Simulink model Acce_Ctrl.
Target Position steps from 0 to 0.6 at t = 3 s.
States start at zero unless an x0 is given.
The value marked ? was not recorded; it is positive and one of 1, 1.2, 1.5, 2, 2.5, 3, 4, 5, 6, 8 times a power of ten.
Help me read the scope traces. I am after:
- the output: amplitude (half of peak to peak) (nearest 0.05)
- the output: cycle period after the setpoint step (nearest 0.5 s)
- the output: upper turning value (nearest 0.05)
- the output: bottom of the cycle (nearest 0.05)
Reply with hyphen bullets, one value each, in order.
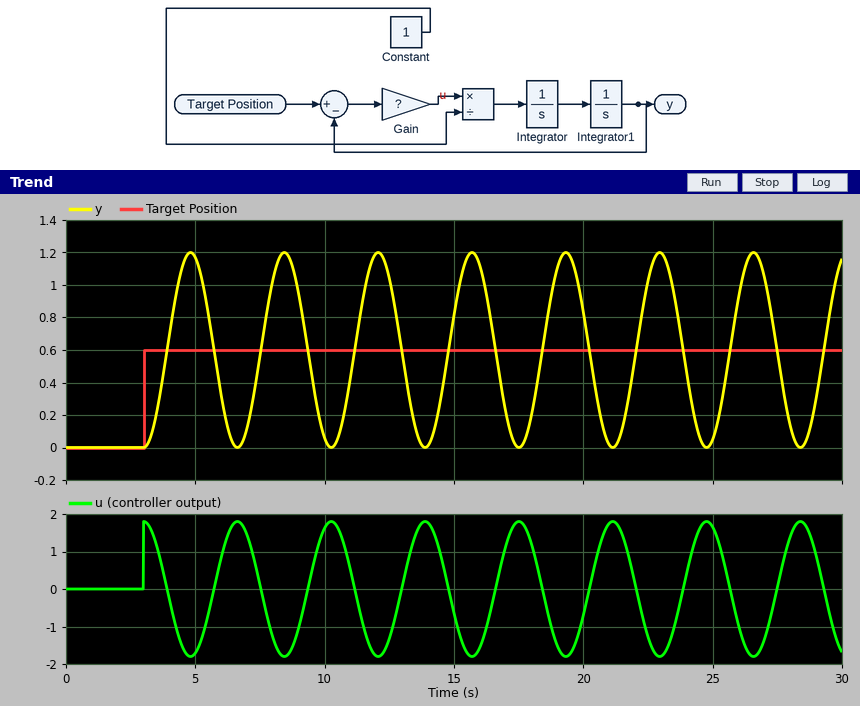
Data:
- 0.60
- 3.5 s
- 1.20
- 0.00
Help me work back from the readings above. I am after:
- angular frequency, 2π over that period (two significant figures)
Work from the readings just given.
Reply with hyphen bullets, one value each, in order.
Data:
- 1.8 rad/s
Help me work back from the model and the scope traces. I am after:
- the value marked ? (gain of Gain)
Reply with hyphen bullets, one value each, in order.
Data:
- 3
